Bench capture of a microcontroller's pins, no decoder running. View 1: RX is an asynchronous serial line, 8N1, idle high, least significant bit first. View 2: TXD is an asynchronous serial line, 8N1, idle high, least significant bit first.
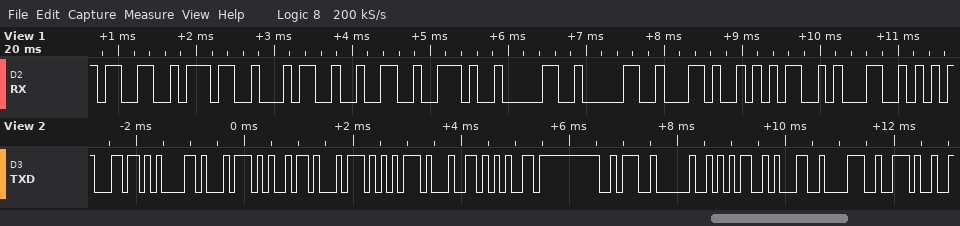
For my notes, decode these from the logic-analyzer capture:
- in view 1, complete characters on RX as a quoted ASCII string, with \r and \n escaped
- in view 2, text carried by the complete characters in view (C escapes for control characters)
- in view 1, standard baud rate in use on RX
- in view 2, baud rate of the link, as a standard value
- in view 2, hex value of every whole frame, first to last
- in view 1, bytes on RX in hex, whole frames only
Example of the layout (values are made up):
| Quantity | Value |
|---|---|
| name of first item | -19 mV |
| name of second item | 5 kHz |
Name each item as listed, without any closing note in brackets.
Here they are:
| Quantity | Value |
|---|---|
| in view 1, complete characters on RX as a quoted ASCII string, with \r and \n escaped | "3742.00,51" |
| in view 2, text carried by the complete characters in view | "latitude: 518." |
| in view 1, standard baud rate in use on RX | 9600 baud |
| in view 2, baud rate of the link, as a standard value | 9600 baud |
| in view 2, hex value of every whole frame, first to last | 0x6C 0x61 0x74 0x69 0x74 0x75 0x64 0x65 0x3A 0x20 0x35 0x31 0x38 0x2E |
| in view 1, bytes on RX in hex, whole frames only | 0x33 0x37 0x34 0x32 0x2E 0x30 0x30 0x2C 0x35 0x31 |
